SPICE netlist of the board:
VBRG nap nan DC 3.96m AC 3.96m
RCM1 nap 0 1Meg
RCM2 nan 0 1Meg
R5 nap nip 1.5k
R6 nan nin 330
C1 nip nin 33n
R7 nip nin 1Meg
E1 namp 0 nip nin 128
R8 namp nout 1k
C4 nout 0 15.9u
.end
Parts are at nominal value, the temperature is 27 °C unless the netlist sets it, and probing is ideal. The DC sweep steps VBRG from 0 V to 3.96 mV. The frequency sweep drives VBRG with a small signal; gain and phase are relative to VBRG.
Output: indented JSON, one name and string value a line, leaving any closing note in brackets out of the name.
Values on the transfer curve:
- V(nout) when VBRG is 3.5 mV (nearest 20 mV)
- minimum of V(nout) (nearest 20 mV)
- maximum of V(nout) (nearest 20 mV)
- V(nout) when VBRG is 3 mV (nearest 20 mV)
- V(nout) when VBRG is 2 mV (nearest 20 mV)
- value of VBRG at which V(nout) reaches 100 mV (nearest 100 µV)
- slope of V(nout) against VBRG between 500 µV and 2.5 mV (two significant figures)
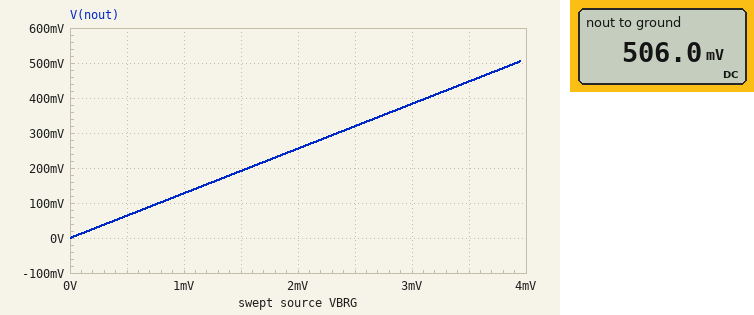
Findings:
{
  "V(nout) when VBRG is 3.5 mV": "440 mV",
  "minimum of V(nout)": "0 V",
  "maximum of V(nout)": "500 mV",
  "V(nout) when VBRG is 3 mV": "380 mV",
  "V(nout) when VBRG is 2 mV": "260 mV",
  "value of VBRG at which V(nout) reaches 100 mV": "800 µV",
  "slope of V(nout) against VBRG between 500 µV and 2.5 mV": "130 V/V"
}
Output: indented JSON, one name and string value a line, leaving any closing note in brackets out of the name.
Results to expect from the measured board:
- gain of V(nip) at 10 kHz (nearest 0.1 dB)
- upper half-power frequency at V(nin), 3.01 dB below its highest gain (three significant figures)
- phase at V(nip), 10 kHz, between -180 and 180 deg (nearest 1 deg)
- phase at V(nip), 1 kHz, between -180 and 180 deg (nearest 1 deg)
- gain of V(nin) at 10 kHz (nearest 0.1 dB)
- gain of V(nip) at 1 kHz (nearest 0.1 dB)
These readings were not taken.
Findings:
{
  "gain of V(nip) at 10 kHz": "-9.5 dB",
  "upper half-power frequency at V(nin), 3.01 dB below its highest gain": "6.20 kHz",
  "phase at V(nip), 10 kHz, between -180 and 180 deg": "-143 deg",
  "phase at V(nip), 1 kHz, between -180 and 180 deg": "-34 deg",
  "gain of V(nin) at 10 kHz": "-9.5 dB",
  "gain of V(nip) at 1 kHz": "-6.4 dB"
}
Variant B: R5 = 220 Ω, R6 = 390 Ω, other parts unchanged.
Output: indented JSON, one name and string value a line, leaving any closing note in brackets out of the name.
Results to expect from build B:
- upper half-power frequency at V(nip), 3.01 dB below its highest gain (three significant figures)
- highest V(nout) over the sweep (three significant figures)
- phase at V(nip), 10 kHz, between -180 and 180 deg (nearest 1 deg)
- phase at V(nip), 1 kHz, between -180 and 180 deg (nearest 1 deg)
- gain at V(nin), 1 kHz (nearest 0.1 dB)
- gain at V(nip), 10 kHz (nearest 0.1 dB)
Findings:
{
  "upper half-power frequency at V(nip), 3.01 dB below its highest gain": "8.61 kHz",
  "highest V(nout) over the sweep": "507 mV",
  "phase at V(nip), 10 kHz, between -180 and 180 deg": "-32 deg",
  "phase at V(nip), 1 kHz, between -180 and 180 deg": "-5 deg",
  "gain at V(nin), 1 kHz": "-6.1 dB",
  "gain at V(nip), 10 kHz": "-9.7 dB"
}
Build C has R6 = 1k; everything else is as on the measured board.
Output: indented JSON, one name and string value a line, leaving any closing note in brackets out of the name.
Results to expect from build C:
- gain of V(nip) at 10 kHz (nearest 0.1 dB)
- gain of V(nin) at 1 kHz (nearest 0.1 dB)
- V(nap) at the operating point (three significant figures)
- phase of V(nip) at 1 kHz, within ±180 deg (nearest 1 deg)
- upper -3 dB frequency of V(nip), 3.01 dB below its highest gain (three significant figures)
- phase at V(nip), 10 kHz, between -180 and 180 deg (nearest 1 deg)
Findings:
{
  "gain of V(nip) at 10 kHz": "-17.3 dB",
  "gain of V(nin) at 1 kHz": "-7.0 dB",
  "V(nap) at the operating point": "1.98 mV",
  "phase of V(nip) at 1 kHz, within ±180 deg": "-33 deg",
  "upper -3 dB frequency of V(nip), 3.01 dB below its highest gain": "2.02 kHz",
  "phase at V(nip), 10 kHz, between -180 and 180 deg": "-125 deg"
}
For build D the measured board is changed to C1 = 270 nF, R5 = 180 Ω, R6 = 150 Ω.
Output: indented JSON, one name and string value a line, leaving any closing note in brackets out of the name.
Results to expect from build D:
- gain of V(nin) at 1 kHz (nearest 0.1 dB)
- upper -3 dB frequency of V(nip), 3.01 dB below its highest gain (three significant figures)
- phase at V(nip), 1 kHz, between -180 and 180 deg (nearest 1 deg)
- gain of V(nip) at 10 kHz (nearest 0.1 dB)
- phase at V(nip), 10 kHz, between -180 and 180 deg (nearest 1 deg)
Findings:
{
  "gain of V(nin) at 1 kHz": "-7.2 dB",
  "upper -3 dB frequency of V(nip), 3.01 dB below its highest gain": "1.80 kHz",
  "phase at V(nip), 1 kHz, between -180 and 180 deg": "-32 deg",
  "gain of V(nip) at 10 kHz": "-20.1 dB",
  "phase at V(nip), 10 kHz, between -180 and 180 deg": "-107 deg"
}
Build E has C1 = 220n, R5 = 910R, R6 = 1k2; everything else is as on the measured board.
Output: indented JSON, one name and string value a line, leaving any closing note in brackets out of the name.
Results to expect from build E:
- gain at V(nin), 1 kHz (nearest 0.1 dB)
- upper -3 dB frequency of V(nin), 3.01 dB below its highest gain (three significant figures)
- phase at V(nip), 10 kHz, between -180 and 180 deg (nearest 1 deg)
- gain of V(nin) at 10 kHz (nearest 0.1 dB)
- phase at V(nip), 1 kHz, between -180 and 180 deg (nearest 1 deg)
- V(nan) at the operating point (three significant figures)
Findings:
{
  "gain at V(nin), 1 kHz": "-15.2 dB",
  "upper -3 dB frequency of V(nin), 3.01 dB below its highest gain": "350 Hz",
  "phase at V(nip), 10 kHz, between -180 and 180 deg": "-12 deg",
  "gain of V(nin) at 10 kHz": "-23.0 dB",
  "phase at V(nip), 1 kHz, between -180 and 180 deg": "-49 deg",
  "V(nan) at the operating point": "-1.98 mV"
}
